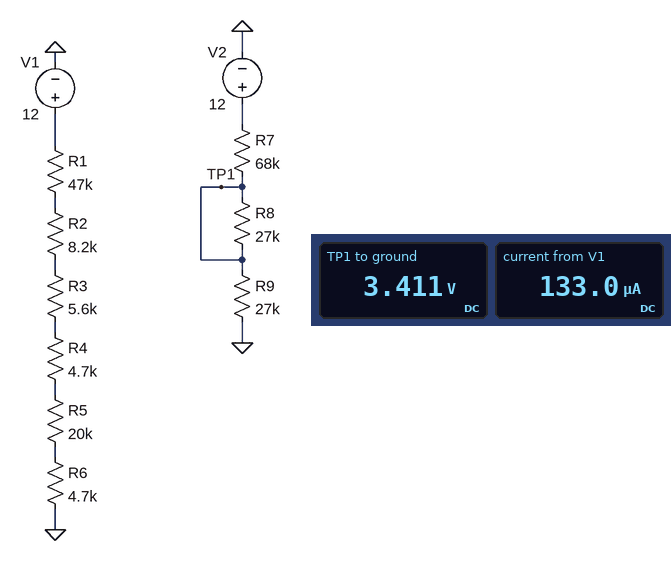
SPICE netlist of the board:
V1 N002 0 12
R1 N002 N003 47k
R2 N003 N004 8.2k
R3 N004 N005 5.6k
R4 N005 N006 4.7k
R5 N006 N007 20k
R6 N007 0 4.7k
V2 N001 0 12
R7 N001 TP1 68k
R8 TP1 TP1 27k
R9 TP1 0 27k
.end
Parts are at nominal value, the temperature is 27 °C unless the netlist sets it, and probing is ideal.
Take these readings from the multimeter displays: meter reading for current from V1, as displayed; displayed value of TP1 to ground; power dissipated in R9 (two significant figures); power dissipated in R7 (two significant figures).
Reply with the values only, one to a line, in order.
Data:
133.0 µA
3.411 V
430 µW
1.1 mW
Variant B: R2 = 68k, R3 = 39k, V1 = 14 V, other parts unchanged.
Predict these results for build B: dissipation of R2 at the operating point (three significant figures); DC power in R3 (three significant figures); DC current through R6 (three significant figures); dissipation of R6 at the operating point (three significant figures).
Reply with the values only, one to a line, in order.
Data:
396 µW
227 µW
76.3 µA
27.4 µW
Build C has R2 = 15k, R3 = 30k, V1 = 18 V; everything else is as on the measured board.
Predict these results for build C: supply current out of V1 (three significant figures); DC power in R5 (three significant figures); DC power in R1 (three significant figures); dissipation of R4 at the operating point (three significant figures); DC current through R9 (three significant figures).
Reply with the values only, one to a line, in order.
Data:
148 µA
440 µW
1.03 mW
103 µW
126 µA
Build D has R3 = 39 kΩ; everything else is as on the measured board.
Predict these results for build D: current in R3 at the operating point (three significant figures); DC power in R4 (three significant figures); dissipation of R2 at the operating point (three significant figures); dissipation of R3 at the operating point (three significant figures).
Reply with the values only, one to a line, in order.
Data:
97.1 µA
44.3 µW
77.3 µW
368 µW
